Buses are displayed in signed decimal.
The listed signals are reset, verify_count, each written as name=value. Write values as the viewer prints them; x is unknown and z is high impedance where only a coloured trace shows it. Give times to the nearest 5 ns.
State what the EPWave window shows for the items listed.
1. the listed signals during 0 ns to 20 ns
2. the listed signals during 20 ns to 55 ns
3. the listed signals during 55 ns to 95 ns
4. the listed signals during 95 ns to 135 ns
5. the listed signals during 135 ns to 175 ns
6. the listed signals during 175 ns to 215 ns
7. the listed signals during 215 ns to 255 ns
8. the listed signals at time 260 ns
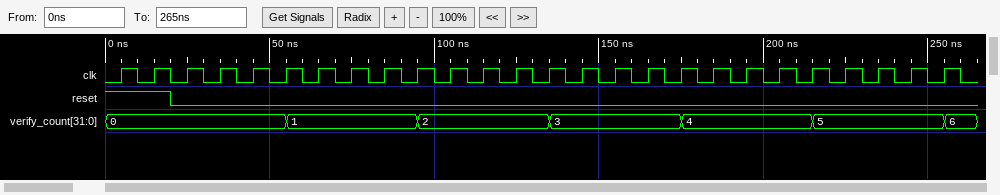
reset=1, verify_count=0
reset=0, verify_count=0
reset=0, verify_count=1
reset=0, verify_count=2
reset=0, verify_count=3
reset=0, verify_count=4
reset=0, verify_count=5
reset=0, verify_count=6
